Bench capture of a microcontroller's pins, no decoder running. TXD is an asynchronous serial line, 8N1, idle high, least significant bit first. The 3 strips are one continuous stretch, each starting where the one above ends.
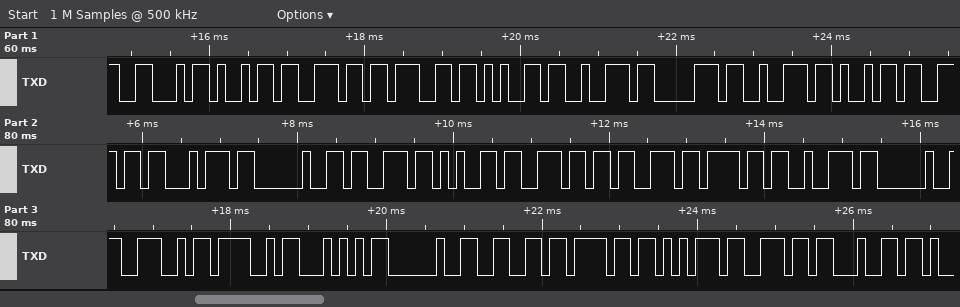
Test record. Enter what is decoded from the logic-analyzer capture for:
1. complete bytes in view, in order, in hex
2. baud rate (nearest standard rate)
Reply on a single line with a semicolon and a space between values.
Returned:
46 69 6E 67 65 72 70 72 69 6E 74 20 73 65 6E 73 6F 72 20 4E 4F 54 20 66 6F 75 6E 64; 9600 baud
